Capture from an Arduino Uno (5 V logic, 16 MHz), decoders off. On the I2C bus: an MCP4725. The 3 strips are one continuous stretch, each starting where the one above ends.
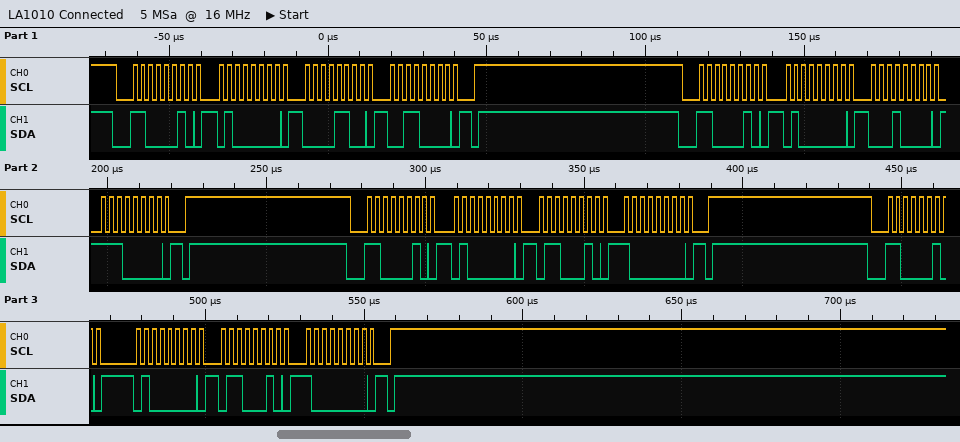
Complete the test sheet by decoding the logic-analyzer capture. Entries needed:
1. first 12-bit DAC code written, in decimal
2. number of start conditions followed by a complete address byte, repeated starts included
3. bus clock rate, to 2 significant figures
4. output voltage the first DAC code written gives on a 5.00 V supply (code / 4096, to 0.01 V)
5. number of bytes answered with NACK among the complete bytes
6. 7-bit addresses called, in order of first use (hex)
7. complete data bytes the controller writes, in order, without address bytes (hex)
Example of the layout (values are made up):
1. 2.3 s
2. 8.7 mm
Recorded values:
1. 195
2. 4
3. 400 kHz
4. 0.24 V
5. 0
6. 0x61
7. 40 0C 30 40 10 E0 40 62 80 40 62 80
